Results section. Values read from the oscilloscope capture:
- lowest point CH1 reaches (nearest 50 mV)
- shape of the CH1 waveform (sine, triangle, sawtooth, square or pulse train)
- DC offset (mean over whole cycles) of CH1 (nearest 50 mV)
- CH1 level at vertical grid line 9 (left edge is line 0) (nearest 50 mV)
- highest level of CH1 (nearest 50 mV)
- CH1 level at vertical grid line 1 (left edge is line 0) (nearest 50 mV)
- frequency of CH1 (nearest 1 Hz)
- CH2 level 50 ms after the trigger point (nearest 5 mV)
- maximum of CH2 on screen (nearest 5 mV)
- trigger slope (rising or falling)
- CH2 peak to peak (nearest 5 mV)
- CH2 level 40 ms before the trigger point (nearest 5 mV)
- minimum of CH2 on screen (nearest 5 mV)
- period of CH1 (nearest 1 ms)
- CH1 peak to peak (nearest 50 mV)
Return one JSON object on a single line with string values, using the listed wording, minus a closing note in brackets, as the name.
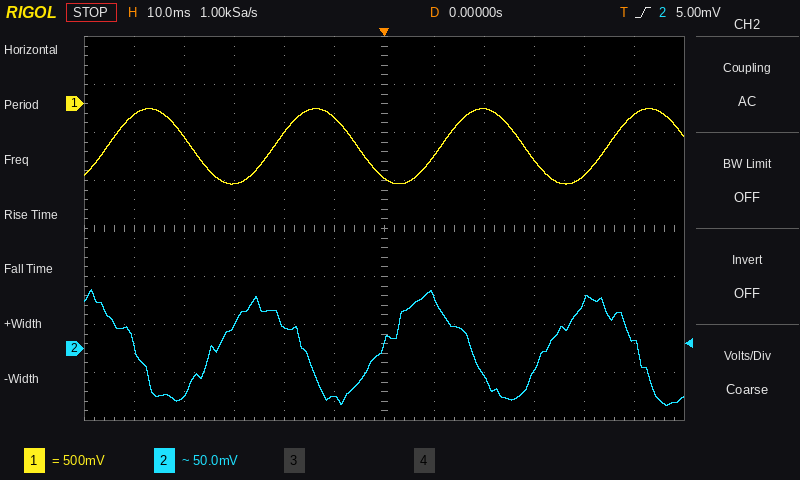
{"lowest point CH1 reaches": "-850 mV", "shape of the CH1 waveform": "sine", "DC offset (mean over whole cycles) of CH1": "-450 mV", "CH1 level at vertical grid line 9 (left edge is line 0)": "-600 mV", "highest level of CH1": "-50 mV", "CH1 level at vertical grid line 1 (left edge is line 0)": "-100 mV", "frequency of CH1": "30 Hz", "CH2 level 50 ms after the trigger point": "5 mV", "maximum of CH2 on screen": "60 mV", "trigger slope": "rising", "CH2 peak to peak": "120 mV", "CH2 level 40 ms before the trigger point": "-50 mV", "minimum of CH2 on screen": "-60 mV", "period of CH1": "33 ms", "CH1 peak to peak": "800 mV"}
